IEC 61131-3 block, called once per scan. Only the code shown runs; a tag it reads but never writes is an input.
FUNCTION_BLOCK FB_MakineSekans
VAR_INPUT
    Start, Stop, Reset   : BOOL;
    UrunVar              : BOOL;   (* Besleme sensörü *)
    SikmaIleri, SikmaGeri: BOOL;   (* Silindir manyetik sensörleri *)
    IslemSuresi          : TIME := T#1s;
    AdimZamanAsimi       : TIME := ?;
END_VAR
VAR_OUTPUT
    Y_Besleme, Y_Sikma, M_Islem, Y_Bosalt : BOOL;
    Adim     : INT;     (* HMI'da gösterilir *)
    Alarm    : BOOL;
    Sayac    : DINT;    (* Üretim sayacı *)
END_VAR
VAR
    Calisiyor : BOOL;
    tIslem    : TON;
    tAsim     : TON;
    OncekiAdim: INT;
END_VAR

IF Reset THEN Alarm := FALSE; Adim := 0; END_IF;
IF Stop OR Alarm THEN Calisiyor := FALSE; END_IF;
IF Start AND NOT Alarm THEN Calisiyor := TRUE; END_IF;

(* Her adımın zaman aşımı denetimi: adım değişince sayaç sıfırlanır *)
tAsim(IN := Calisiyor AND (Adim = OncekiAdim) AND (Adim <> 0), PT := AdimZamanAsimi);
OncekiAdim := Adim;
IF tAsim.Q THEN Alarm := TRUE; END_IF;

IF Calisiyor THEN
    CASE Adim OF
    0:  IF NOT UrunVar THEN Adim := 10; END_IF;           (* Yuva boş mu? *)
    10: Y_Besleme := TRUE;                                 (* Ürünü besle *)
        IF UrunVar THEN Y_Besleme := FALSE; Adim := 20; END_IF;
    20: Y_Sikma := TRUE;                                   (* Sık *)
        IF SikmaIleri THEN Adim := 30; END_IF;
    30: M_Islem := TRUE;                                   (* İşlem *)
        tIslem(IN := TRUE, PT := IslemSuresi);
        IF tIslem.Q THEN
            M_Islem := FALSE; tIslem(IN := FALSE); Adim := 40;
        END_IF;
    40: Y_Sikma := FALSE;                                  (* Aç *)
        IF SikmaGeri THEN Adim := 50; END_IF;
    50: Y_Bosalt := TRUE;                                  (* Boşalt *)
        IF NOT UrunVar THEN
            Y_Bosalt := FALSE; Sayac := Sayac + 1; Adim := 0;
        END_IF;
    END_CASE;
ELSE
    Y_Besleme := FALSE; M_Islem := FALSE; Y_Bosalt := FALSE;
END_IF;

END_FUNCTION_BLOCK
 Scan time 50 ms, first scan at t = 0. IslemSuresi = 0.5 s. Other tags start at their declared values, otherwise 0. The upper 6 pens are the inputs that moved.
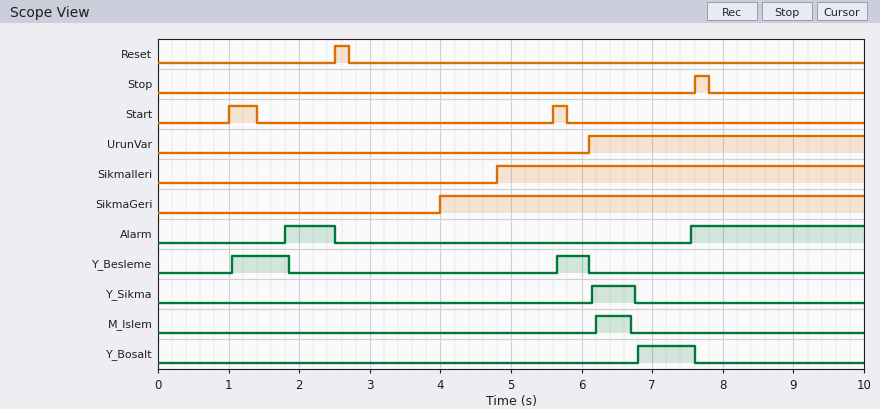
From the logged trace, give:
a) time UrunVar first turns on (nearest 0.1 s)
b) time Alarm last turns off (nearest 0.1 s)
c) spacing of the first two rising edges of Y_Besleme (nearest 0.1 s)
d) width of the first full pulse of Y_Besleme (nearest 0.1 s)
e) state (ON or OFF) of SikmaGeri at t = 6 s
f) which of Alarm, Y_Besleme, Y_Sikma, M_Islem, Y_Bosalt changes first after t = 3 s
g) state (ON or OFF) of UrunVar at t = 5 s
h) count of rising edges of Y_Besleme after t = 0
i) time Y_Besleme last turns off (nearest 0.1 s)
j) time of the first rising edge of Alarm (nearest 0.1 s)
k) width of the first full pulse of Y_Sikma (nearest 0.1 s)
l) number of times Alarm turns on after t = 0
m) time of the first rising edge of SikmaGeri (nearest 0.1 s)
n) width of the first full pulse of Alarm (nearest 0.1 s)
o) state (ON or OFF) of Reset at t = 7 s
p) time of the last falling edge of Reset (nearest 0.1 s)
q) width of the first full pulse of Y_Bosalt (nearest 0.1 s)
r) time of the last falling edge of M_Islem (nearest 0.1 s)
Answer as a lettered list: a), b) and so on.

a) 6.1 s
b) 2.5 s
c) 4.6 s
d) 0.8 s
e) ON
f) Y_Besleme
g) OFF
h) 2
i) 6.1 s
j) 1.8 s
k) 0.6 s
l) 2
m) 4.0 s
n) 0.7 s
o) OFF
p) 2.7 s
q) 0.8 s
r) 6.7 s
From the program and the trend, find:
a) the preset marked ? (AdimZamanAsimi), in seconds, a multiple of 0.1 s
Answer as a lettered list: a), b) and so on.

a) 0.7 s
